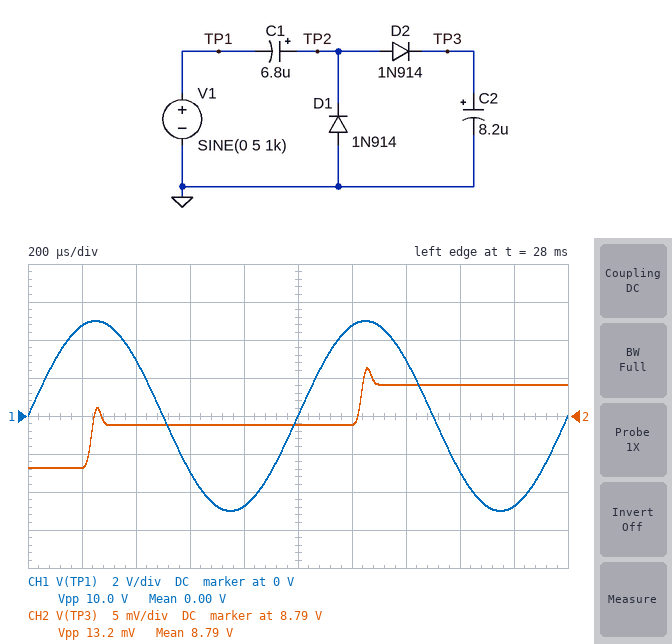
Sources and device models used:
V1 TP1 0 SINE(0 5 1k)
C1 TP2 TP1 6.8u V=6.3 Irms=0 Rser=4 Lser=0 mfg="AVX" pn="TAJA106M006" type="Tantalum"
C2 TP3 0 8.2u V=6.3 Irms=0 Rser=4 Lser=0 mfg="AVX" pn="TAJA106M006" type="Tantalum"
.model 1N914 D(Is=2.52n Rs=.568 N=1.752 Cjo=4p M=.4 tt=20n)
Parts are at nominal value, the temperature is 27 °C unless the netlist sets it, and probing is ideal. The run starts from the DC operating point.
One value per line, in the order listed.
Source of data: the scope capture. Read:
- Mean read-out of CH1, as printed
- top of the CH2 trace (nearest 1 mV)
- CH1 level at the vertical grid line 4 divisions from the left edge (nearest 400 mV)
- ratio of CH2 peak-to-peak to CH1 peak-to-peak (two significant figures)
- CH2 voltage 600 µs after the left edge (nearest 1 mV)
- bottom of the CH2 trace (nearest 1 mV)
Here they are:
0.00 V
8.796 V
-4.8 V
0.0013
8.789 V
8.783 V
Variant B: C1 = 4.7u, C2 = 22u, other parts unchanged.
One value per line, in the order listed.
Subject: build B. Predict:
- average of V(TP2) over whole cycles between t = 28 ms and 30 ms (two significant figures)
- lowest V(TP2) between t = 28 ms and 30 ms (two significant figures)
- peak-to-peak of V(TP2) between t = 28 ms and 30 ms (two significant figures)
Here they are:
4.3 V
-680 mV
9.9 V
